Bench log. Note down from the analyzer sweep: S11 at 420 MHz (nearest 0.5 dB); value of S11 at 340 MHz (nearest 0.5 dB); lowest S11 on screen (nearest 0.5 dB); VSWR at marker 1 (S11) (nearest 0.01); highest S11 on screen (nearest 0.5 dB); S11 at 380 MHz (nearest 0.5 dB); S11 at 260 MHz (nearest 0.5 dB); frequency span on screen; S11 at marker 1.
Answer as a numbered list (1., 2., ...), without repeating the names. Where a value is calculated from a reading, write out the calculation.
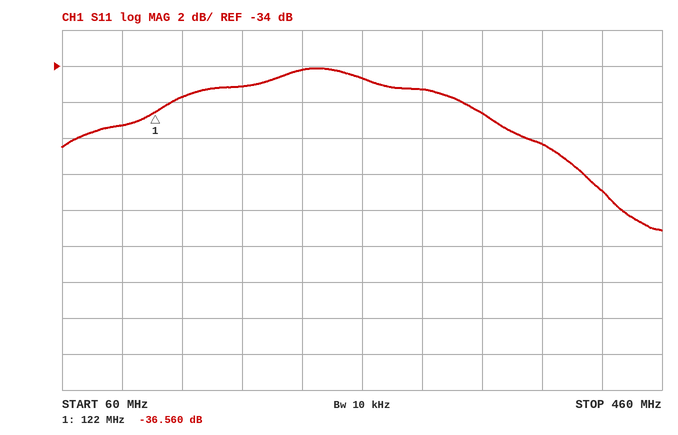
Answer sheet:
1. -41.0 dB
2. -36.5 dB
3. -43.0 dB
4. (1 + 0.0149)/(1 − 0.0149) ≈ 1.03
5. -34.0 dB
6. -38.5 dB
7. -34.5 dB
8. 400 MHz
9. -36.560 dB
